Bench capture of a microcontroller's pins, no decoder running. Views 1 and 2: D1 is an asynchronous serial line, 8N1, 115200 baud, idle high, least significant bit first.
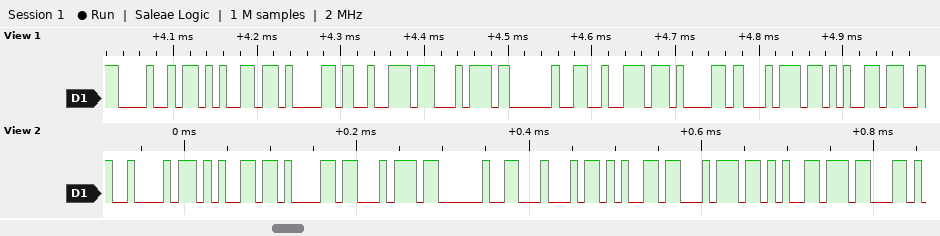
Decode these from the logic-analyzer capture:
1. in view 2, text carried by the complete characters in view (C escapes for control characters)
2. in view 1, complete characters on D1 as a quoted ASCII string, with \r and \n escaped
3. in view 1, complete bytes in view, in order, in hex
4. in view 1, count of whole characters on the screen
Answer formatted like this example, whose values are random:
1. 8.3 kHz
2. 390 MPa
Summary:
1. "Beat Detec"
2. "Heart rate"
3. 0x48 0x65 0x61 0x72 0x74 0x20 0x72 0x61 0x74 0x65
4. 10
